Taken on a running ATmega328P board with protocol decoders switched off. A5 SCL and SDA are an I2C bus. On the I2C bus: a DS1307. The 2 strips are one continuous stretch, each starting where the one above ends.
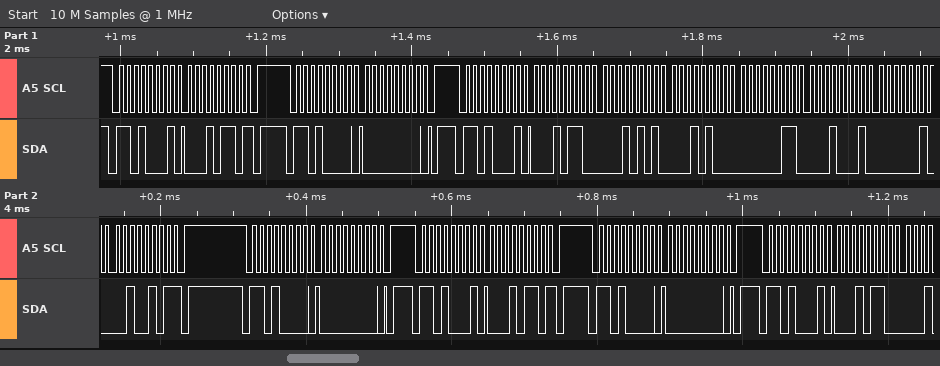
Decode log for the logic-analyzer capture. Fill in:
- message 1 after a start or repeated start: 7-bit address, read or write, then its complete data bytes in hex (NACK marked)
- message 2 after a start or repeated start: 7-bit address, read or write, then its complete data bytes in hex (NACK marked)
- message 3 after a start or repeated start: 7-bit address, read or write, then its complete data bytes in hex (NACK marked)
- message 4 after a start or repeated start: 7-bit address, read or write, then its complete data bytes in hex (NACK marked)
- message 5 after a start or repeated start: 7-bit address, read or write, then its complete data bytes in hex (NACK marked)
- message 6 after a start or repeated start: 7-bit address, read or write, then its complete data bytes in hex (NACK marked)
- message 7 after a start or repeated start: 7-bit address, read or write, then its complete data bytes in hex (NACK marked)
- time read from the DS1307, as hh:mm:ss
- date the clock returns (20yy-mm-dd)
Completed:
0x68 read: 16 NACK
0x68 write: 00
0x68 read: 16 15 14 03 11 02 25 NACK
0x68 write: 00
0x68 read: 16 NACK
0x68 write: 00
0x68 read: 16
14:15:16
2025-02-11
